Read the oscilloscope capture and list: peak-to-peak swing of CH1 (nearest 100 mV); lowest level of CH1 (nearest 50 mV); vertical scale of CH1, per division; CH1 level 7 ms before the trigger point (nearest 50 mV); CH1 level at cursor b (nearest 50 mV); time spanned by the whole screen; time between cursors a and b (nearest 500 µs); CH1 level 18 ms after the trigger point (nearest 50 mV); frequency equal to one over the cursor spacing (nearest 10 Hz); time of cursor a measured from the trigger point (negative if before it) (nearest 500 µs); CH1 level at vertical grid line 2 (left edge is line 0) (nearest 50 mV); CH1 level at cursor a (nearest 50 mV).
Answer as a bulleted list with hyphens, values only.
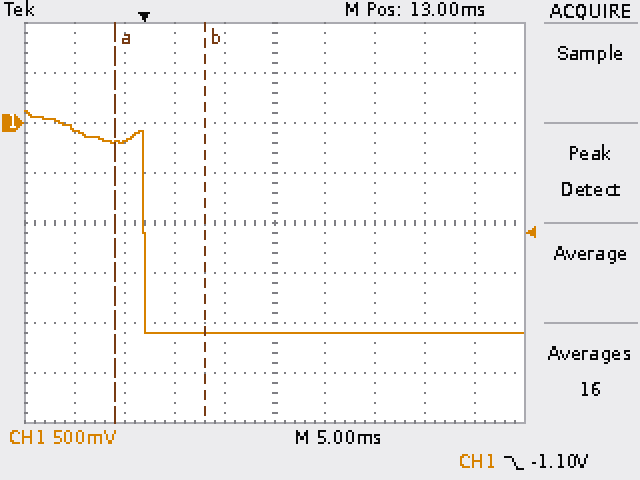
- 2.20 V
- -2.10 V
- 500 mV
- -50 mV
- -2.10 V
- 50 ms
- 9.0 ms
- -2.10 V
- 110 Hz
- -3.0 ms
- -200 mV
- -200 mV
